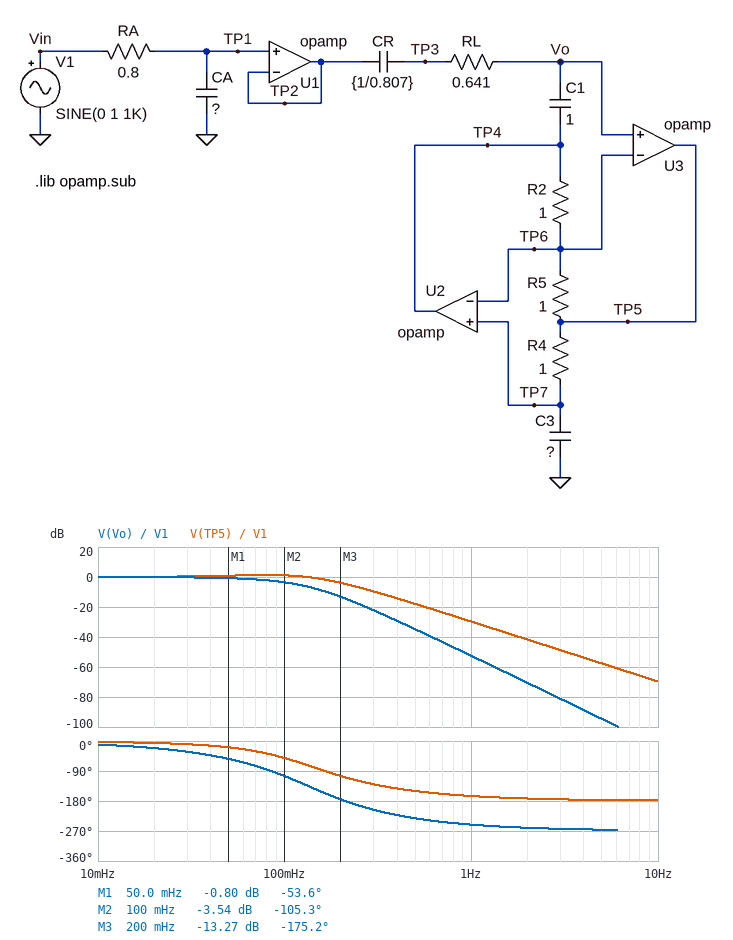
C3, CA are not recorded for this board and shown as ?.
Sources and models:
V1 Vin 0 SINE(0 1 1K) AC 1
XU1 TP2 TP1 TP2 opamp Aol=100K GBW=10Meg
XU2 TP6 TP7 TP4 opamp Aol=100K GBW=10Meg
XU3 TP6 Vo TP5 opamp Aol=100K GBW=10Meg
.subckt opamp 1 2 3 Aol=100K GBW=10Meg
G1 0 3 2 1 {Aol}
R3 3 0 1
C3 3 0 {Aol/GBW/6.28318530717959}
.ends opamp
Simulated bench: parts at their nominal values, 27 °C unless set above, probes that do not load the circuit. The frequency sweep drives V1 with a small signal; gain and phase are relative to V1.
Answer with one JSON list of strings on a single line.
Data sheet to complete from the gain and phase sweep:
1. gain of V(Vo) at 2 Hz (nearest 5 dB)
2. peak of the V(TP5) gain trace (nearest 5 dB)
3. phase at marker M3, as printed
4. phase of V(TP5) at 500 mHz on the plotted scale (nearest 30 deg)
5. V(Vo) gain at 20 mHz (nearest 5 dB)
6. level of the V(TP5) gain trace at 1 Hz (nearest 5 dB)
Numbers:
["-70 dB", "0 dB", "-175.2 deg", "-150 deg", "0 dB", "-30 dB"]
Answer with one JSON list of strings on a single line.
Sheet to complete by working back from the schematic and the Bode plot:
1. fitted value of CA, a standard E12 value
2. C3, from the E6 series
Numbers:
["1.5 F", "2.2 F"]
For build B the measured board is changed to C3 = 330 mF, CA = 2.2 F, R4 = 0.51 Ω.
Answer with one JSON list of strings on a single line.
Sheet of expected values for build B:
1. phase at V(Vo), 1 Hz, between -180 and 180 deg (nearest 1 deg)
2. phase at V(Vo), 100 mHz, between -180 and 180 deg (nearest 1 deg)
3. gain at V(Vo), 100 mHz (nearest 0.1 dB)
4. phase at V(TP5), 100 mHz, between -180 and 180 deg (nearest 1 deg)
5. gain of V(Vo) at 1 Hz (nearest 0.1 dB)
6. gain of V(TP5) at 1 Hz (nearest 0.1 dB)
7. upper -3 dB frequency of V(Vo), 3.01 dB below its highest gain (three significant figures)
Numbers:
["110 deg", "-53 deg", "-3.1 dB", "-47 deg", "-31.5 dB", "-28.2 dB", "97.2 mHz"]
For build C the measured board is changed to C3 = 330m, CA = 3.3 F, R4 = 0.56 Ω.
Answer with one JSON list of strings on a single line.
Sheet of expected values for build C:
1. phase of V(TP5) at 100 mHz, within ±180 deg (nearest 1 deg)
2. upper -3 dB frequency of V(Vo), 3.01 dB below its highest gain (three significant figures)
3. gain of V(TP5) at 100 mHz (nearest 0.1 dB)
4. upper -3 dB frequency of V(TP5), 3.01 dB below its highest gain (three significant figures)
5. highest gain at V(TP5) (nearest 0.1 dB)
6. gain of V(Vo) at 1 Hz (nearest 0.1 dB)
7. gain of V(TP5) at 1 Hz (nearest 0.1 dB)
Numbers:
["-58 deg", "62.3 mHz", "-5.3 dB", "62.6 mHz", "0 dB", "-36.0 dB", "-32.3 dB"]
